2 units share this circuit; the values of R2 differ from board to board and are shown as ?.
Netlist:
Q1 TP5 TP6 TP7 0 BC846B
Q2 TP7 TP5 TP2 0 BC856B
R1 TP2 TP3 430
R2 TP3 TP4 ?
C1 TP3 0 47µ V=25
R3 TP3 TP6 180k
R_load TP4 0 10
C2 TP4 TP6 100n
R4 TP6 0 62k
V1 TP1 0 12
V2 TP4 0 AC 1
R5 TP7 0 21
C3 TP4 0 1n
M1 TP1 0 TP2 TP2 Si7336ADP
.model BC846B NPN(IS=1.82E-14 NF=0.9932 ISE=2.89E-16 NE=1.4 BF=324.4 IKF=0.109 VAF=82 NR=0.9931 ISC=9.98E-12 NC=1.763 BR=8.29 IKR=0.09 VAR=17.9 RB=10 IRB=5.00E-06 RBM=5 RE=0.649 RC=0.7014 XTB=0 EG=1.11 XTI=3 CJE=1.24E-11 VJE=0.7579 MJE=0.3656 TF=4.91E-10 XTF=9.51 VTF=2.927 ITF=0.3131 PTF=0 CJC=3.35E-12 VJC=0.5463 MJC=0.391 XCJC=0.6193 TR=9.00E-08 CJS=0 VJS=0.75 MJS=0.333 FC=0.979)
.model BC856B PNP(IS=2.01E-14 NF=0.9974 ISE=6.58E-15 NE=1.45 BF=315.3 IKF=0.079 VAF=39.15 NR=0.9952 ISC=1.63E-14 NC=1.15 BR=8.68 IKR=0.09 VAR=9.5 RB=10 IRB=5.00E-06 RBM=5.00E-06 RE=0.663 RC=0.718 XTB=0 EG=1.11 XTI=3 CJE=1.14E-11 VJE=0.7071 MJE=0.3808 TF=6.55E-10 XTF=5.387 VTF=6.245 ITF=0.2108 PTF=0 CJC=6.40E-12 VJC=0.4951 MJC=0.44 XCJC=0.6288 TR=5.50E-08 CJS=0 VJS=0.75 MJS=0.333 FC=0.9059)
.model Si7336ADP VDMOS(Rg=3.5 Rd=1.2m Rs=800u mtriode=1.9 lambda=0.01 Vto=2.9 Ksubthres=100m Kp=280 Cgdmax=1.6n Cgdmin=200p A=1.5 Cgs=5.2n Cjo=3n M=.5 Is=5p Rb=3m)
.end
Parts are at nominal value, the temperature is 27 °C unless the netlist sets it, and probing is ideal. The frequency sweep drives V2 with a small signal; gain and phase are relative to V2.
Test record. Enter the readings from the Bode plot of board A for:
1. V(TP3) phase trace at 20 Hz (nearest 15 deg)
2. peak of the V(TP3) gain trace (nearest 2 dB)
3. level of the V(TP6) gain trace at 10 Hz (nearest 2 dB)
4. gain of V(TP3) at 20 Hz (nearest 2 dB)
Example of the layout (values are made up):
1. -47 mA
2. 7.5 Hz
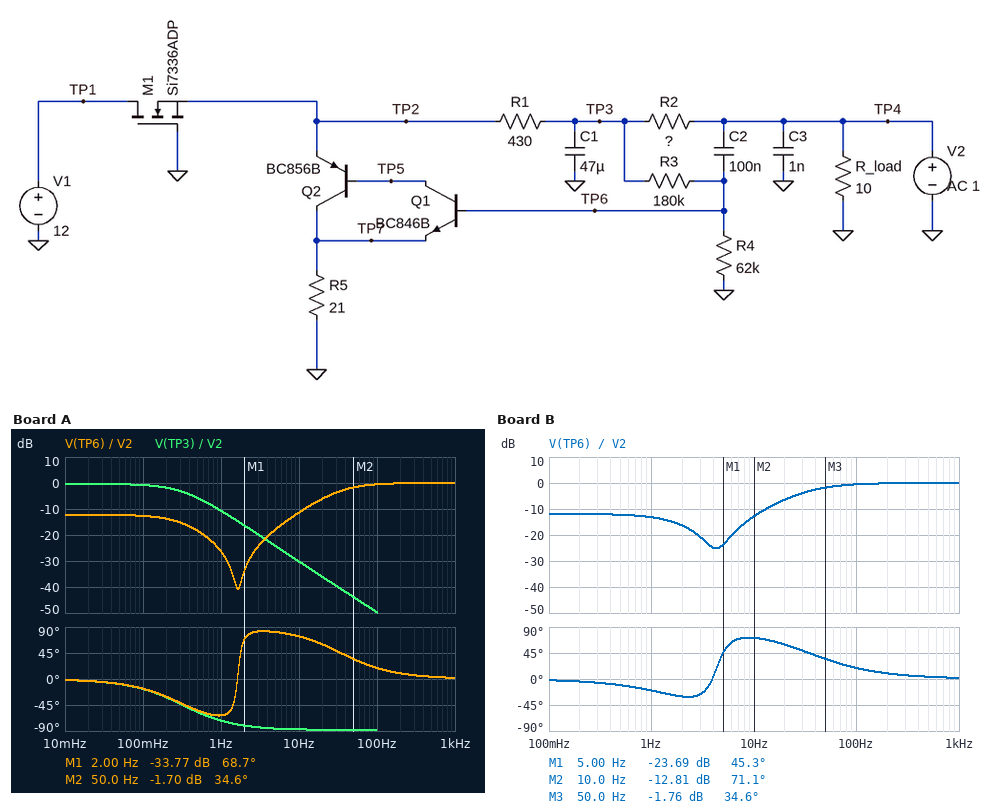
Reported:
1. -90 deg
2. 0 dB
3. -12 dB
4. -36 dB
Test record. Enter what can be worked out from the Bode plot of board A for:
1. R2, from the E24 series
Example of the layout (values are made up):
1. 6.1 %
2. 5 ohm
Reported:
1. 11 kΩ
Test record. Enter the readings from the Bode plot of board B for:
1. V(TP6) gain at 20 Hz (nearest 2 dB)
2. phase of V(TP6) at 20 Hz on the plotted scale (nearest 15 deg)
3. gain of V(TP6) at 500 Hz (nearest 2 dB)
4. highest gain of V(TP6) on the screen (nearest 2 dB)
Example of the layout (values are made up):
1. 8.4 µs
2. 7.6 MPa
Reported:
1. -6 dB
2. 60 deg
3. 0 dB
4. 0 dB
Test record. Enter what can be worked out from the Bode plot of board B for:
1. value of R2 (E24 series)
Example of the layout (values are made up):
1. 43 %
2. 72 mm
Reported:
1. 1.6 kΩ
